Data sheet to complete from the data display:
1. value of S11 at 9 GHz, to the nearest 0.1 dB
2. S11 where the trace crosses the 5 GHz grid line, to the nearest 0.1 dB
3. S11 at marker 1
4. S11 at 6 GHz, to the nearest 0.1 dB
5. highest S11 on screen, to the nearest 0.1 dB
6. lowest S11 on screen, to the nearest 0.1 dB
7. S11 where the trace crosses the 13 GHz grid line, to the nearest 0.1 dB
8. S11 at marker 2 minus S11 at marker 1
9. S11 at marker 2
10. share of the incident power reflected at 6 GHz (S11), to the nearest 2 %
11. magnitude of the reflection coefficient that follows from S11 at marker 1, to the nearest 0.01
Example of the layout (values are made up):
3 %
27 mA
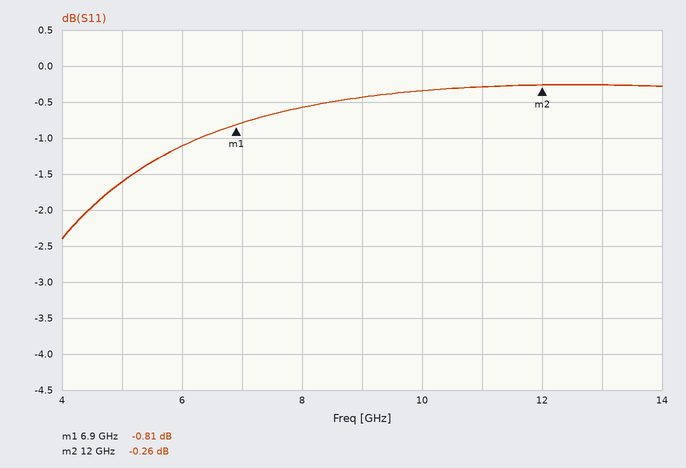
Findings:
-0.4 dB
-1.6 dB
-0.81 dB
-1.1 dB
-0.3 dB
-2.4 dB
-0.3 dB
0.55 dB
-0.26 dB
78 %
0.91
